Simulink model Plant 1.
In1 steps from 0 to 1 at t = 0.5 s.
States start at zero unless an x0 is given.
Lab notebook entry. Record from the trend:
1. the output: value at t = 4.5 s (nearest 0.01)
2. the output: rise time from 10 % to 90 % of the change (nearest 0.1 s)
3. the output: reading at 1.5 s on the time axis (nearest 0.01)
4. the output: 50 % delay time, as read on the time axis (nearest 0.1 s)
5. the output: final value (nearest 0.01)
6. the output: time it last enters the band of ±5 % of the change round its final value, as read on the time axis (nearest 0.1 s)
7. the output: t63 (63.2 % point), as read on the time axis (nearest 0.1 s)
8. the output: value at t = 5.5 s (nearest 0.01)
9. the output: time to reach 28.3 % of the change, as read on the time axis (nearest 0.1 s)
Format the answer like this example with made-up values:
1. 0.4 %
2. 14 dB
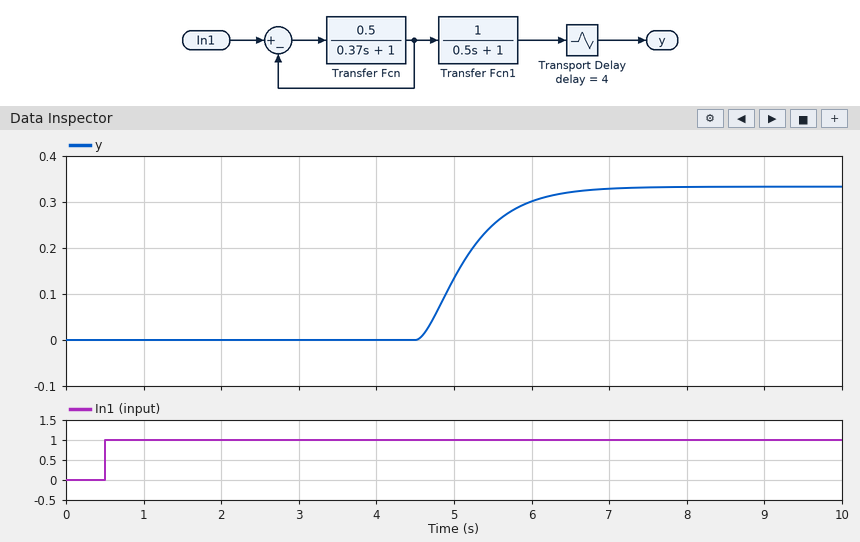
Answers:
1. 0.00
2. 1.3 s
3. 0.00
4. 5.1 s
5. 0.33
6. 6.3 s
7. 5.3 s
8. 0.25
9. 4.9 s
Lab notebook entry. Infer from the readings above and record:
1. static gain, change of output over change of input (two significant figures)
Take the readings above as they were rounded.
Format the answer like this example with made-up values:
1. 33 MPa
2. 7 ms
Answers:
1. 0.33
